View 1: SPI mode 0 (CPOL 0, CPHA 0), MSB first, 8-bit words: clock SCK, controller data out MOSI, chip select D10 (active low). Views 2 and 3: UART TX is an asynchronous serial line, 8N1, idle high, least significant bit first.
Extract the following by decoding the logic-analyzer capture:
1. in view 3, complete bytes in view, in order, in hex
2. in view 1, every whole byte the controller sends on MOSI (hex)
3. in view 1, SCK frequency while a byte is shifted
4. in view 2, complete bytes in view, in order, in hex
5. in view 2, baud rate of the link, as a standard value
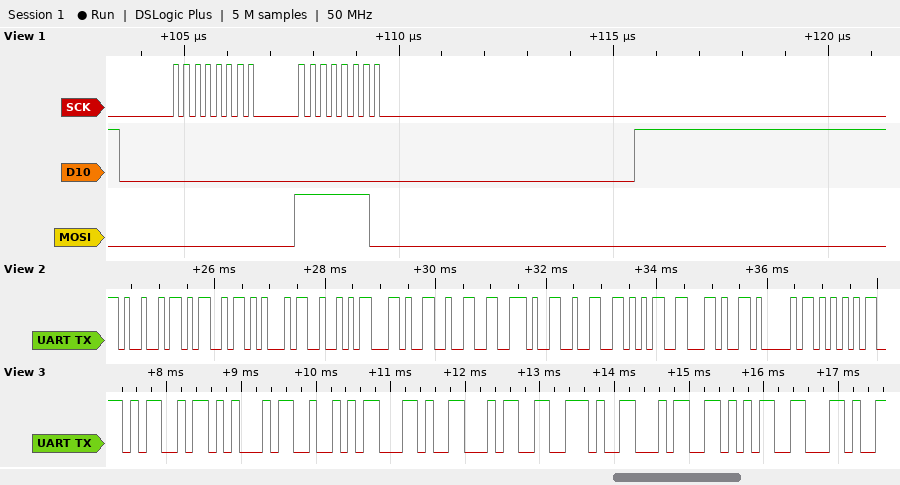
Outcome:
4D 45 52 2C 34 2E 34 35 2C
00 FE
4 MHz
49 4D 45 52 2C 32 2E 32 35 2C 41 55
9600 baud
